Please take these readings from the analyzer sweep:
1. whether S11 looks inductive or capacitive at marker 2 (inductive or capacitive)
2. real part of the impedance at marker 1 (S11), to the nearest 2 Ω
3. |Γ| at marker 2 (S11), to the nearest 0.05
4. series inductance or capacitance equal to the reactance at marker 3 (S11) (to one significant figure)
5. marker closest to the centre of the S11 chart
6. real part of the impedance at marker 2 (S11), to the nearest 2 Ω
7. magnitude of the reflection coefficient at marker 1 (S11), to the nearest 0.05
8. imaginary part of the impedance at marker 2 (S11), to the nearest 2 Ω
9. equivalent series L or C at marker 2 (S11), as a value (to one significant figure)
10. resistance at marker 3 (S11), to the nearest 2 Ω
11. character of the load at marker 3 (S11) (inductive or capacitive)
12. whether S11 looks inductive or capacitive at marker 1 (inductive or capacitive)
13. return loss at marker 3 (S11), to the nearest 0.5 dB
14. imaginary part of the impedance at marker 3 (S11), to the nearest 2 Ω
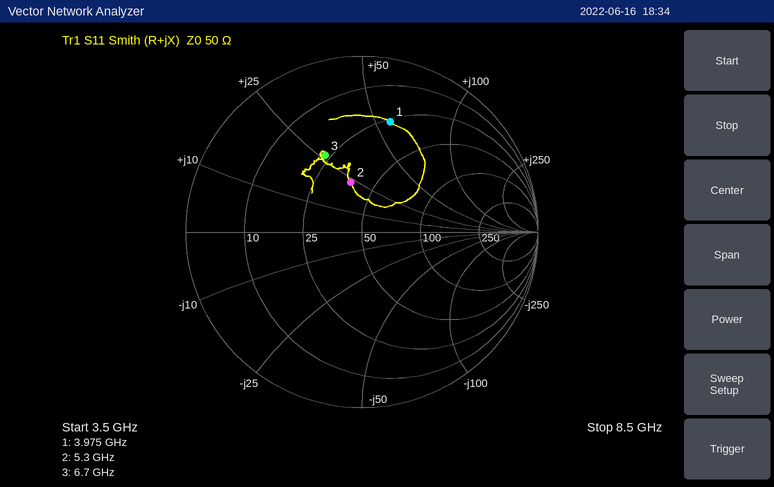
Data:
inductive
26 Ω
0.30
600 pH
marker 2
38 Ω
0.65
+24 Ω
700 pH
24 Ω
inductive
inductive
6.5 dB
+26 Ω
